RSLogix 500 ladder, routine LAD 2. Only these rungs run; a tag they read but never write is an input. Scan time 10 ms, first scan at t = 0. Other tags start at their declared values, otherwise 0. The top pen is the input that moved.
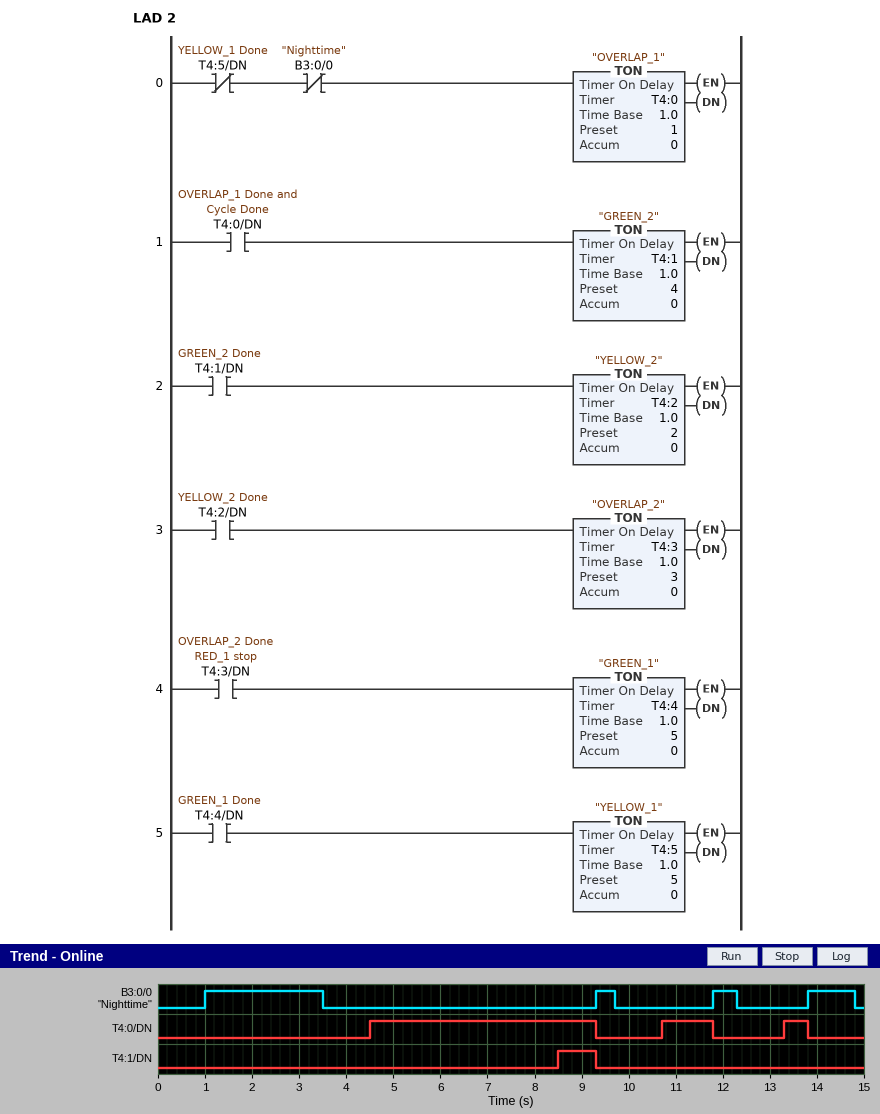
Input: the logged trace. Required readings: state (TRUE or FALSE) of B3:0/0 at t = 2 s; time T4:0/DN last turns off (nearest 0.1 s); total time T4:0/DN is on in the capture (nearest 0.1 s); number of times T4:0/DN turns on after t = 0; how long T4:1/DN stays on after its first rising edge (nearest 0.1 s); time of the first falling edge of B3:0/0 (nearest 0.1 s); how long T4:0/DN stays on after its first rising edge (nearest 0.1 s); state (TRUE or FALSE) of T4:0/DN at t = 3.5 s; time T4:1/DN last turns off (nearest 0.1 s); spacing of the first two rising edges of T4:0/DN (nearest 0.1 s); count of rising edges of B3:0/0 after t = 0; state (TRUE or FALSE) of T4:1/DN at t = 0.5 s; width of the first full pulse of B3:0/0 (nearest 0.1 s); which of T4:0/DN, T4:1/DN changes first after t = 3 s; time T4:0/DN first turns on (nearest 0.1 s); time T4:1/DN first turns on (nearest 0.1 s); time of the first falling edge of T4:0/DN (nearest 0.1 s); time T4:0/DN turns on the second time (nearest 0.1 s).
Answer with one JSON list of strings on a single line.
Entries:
["TRUE", "13.8 s", "6.4 s", "3", "0.8 s", "3.5 s", "4.8 s", "FALSE", "9.3 s", "6.2 s", "4", "FALSE", "2.5 s", "T4:0/DN", "4.5 s", "8.5 s", "9.3 s", "10.7 s"]
